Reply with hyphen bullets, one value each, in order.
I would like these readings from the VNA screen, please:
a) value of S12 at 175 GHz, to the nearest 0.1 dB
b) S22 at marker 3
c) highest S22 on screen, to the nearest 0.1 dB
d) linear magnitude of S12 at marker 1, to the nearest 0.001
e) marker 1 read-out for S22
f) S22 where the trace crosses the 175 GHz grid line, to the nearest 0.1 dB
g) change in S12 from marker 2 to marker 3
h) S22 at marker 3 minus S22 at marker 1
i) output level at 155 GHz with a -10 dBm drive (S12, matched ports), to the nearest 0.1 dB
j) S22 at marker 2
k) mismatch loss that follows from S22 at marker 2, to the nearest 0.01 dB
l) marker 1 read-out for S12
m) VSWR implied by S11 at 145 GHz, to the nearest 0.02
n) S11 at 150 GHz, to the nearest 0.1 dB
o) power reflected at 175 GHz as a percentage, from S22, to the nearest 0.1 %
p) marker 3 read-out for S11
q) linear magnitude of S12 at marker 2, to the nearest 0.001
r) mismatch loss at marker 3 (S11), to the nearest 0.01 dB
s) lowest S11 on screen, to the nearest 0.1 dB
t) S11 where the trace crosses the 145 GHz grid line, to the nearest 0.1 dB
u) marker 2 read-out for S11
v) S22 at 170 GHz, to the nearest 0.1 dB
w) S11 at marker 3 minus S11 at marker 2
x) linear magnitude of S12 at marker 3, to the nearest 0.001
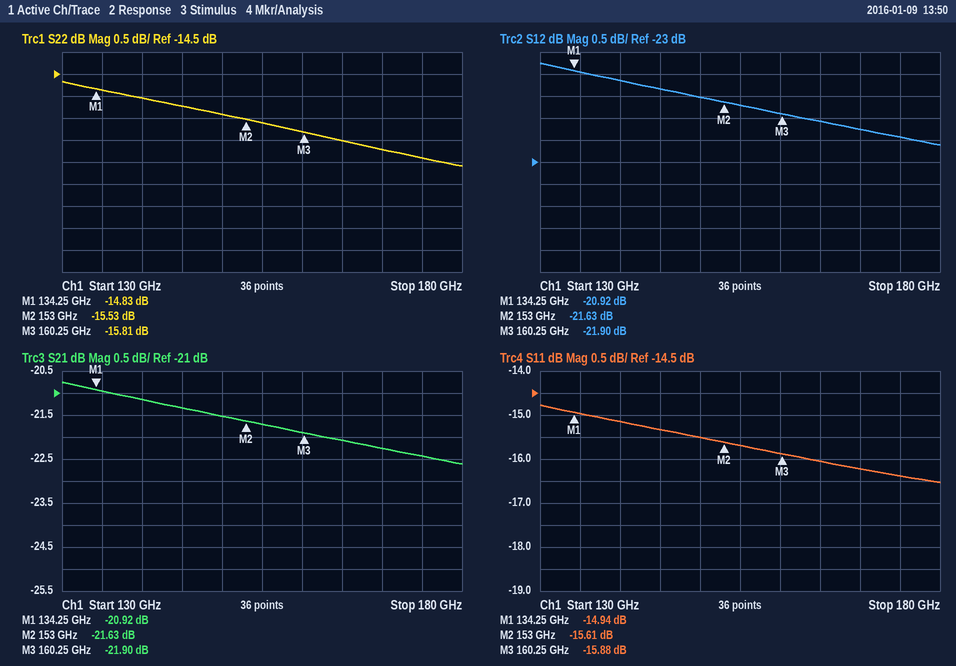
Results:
- -22.4 dB
- -15.81 dB
- -14.7 dB
- 0.090
- -14.83 dB
- -16.4 dB
- -0.27 dB
- -0.98 dB
- -31.7 dBm
- -15.53 dB
- 0.12 dB
- -20.92 dB
- 1.42
- -15.5 dB
- 2.3 %
- -15.88 dB
- 0.083
- 0.11 dB
- -16.5 dB
- -15.3 dB
- -15.61 dB
- -16.2 dB
- -0.27 dB
- 0.080
